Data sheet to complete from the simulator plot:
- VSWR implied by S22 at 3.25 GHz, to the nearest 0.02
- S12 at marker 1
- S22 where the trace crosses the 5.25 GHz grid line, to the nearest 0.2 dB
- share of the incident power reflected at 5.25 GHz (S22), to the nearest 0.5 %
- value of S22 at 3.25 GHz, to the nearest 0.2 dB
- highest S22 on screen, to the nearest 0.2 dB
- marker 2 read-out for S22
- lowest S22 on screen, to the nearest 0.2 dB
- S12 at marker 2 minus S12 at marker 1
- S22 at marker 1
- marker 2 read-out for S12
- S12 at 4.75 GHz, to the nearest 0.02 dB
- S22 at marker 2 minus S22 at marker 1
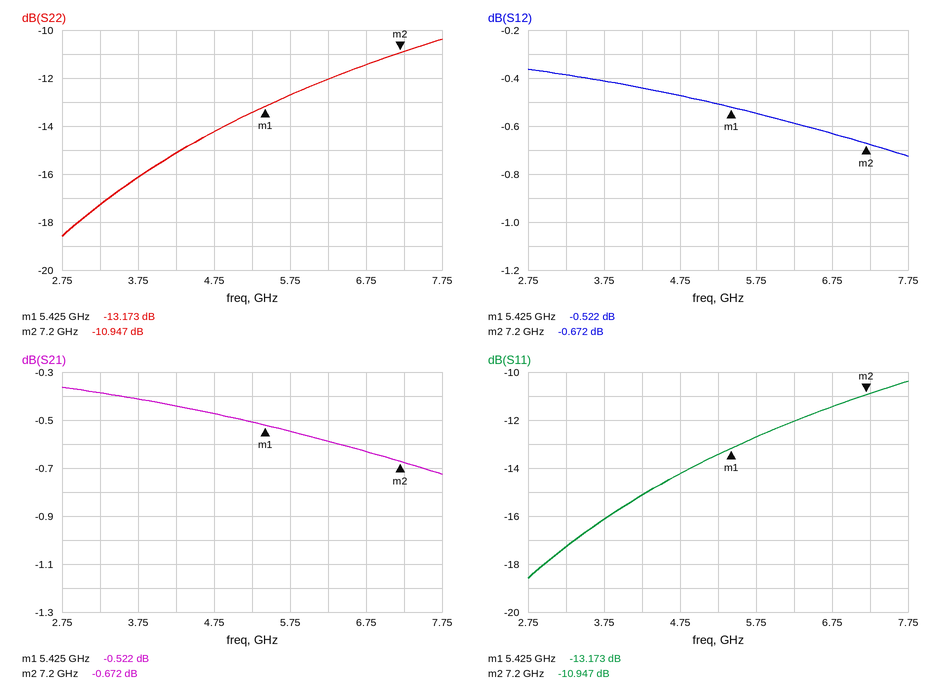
1.32
-0.522 dB
-13.4 dB
4.5 %
-17.2 dB
-10.4 dB
-10.947 dB
-18.6 dB
-0.150 dB
-13.173 dB
-0.672 dB
-0.48 dB
2.226 dB
